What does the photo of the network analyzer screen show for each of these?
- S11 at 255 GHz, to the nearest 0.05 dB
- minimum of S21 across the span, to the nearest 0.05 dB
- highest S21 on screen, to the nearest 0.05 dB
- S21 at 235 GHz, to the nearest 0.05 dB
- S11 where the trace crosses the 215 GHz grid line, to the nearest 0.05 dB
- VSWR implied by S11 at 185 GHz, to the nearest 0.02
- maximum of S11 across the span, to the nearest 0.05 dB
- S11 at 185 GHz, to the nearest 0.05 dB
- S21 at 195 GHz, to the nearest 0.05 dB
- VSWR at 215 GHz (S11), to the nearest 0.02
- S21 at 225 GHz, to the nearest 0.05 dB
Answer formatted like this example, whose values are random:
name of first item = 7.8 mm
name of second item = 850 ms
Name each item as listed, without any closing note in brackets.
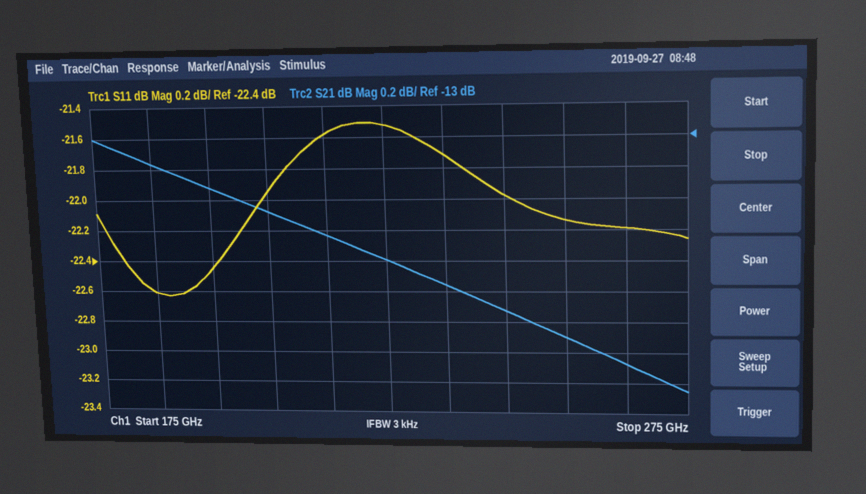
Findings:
S11 at 255 GHz, to the nearest 0.05 dB = -22.15 dB
minimum of S21 across the span, to the nearest 0.05 dB = -14.65 dB
highest S21 on screen, to the nearest 0.05 dB = -13.00 dB
S21 at 235 GHz, to the nearest 0.05 dB = -13.95 dB
S11 where the trace crosses the 215 GHz grid line, to the nearest 0.05 dB = -21.60 dB
VSWR implied by S11 at 185 GHz, to the nearest 0.02 = 1.16
maximum of S11 across the span, to the nearest 0.05 dB = -21.50 dB
S11 at 185 GHz, to the nearest 0.05 dB = -22.60 dB
S21 at 195 GHz, to the nearest 0.05 dB = -13.30 dB
VSWR at 215 GHz (S11), to the nearest 0.02 = 1.18
S21 at 225 GHz, to the nearest 0.05 dB = -13.80 dB
